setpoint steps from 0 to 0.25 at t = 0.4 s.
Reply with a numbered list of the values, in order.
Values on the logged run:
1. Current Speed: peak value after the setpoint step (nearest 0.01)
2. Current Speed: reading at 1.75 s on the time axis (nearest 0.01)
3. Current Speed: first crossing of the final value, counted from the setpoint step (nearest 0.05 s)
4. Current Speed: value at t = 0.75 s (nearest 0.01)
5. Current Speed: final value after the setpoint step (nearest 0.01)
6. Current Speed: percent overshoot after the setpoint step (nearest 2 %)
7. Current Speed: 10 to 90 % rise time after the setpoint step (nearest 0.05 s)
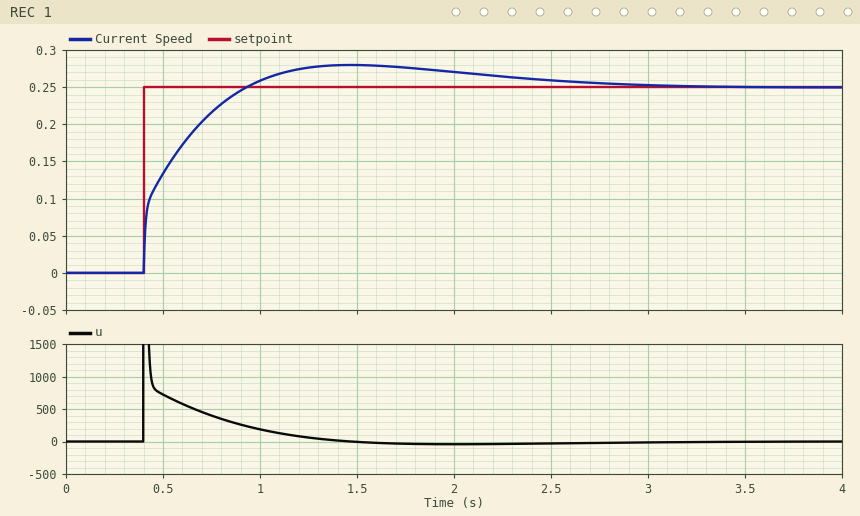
1. 0.28
2. 0.28
3. 0.55 s
4. 0.22
5. 0.25
6. 12 %
7. 0.40 s
